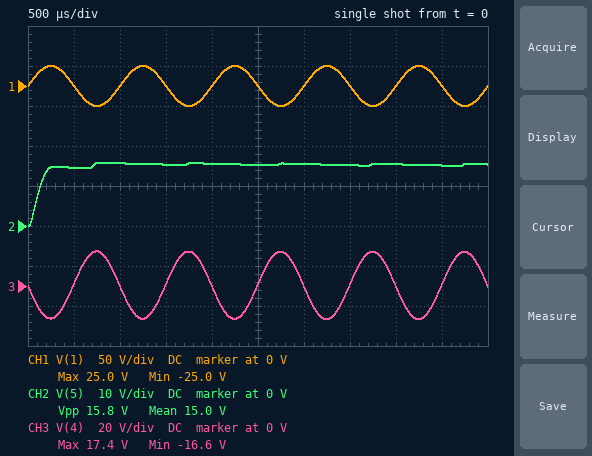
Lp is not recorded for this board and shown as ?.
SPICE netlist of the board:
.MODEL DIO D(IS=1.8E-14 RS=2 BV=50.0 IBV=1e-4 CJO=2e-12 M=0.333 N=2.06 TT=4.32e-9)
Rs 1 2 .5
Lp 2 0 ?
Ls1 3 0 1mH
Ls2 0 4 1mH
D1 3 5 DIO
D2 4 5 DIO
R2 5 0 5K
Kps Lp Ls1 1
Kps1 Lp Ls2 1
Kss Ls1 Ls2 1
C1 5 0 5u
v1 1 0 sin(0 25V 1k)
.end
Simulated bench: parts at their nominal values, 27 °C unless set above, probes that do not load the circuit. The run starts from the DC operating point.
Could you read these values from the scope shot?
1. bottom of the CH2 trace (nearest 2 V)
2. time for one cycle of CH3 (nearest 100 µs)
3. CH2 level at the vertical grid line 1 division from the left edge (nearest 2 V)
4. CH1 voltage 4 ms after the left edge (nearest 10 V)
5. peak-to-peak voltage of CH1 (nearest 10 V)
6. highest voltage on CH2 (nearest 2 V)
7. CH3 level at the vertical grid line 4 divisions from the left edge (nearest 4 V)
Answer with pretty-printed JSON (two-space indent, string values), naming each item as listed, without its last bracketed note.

{
  "bottom of the CH2 trace": "0 V",
  "time for one cycle of CH3": "1.0 ms",
  "CH2 level at the vertical grid line 1 division from the left edge": "14 V",
  "CH1 voltage 4 ms after the left edge": "0 V",
  "peak-to-peak voltage of CH1": "50 V",
  "highest voltage on CH2": "16 V",
  "CH3 level at the vertical grid line 4 divisions from the left edge": "0 V"
}
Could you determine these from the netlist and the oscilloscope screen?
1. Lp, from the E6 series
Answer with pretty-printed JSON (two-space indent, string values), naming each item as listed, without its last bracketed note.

{
  "Lp, from the E6 series": "2.2 mH"
}
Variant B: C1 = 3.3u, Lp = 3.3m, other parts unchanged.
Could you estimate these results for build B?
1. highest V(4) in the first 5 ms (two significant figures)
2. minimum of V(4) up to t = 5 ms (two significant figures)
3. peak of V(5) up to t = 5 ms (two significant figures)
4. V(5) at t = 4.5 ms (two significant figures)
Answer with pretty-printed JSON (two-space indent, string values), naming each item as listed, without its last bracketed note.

{
  "highest V(4) in the first 5 ms": "14 V",
  "minimum of V(4) up to t = 5 ms": "-14 V",
  "peak of V(5) up to t = 5 ms": "13 V",
  "V(5) at t = 4.5 ms": "12 V"
}
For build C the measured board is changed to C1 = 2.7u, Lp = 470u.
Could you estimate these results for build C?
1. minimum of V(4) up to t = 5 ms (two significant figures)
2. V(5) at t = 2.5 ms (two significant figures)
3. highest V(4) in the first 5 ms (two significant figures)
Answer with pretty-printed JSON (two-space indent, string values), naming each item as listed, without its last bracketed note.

{
  "minimum of V(4) up to t = 5 ms": "-31 V",
  "V(5) at t = 2.5 ms": "24 V",
  "highest V(4) in the first 5 ms": "32 V"
}
